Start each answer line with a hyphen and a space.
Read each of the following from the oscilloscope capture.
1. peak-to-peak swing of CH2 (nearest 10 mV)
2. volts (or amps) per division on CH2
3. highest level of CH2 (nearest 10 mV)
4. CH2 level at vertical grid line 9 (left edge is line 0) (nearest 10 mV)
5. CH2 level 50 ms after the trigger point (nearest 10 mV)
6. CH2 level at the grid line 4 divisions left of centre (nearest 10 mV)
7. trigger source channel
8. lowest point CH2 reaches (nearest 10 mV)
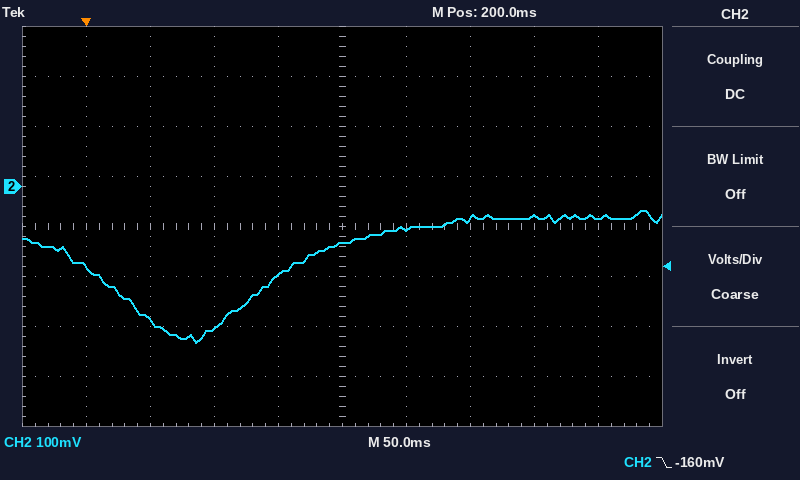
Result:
- 260 mV
- 100 mV
- -50 mV
- -60 mV
- -270 mV
- -160 mV
- CH2
- -310 mV
